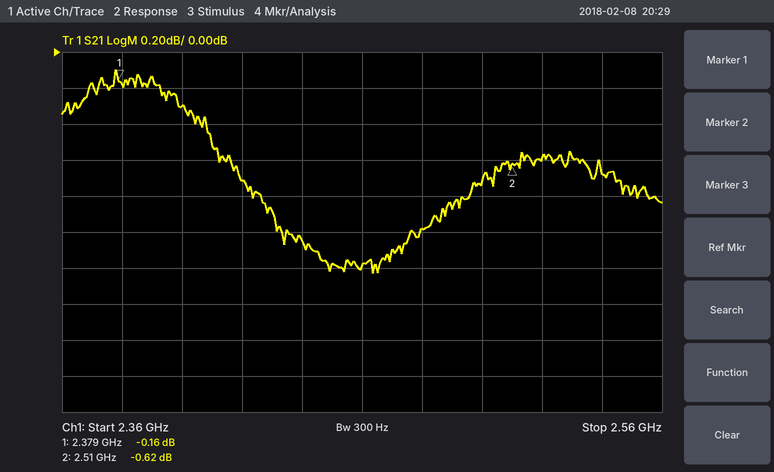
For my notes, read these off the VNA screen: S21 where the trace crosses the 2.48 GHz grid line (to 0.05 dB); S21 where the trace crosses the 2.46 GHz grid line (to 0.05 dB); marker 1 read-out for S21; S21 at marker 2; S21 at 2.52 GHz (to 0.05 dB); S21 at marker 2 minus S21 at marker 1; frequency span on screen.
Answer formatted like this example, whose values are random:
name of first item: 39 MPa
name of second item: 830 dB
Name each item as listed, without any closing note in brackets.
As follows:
S21 where the trace crosses the 2.48 GHz grid line: -1.00 dB
S21 where the trace crosses the 2.46 GHz grid line: -1.20 dB
marker 1 read-out for S21: -0.16 dB
S21 at marker 2: -0.62 dB
S21 at 2.52 GHz: -0.60 dB
S21 at marker 2 minus S21 at marker 1: -0.46 dB
frequency span on screen: 200 MHz
